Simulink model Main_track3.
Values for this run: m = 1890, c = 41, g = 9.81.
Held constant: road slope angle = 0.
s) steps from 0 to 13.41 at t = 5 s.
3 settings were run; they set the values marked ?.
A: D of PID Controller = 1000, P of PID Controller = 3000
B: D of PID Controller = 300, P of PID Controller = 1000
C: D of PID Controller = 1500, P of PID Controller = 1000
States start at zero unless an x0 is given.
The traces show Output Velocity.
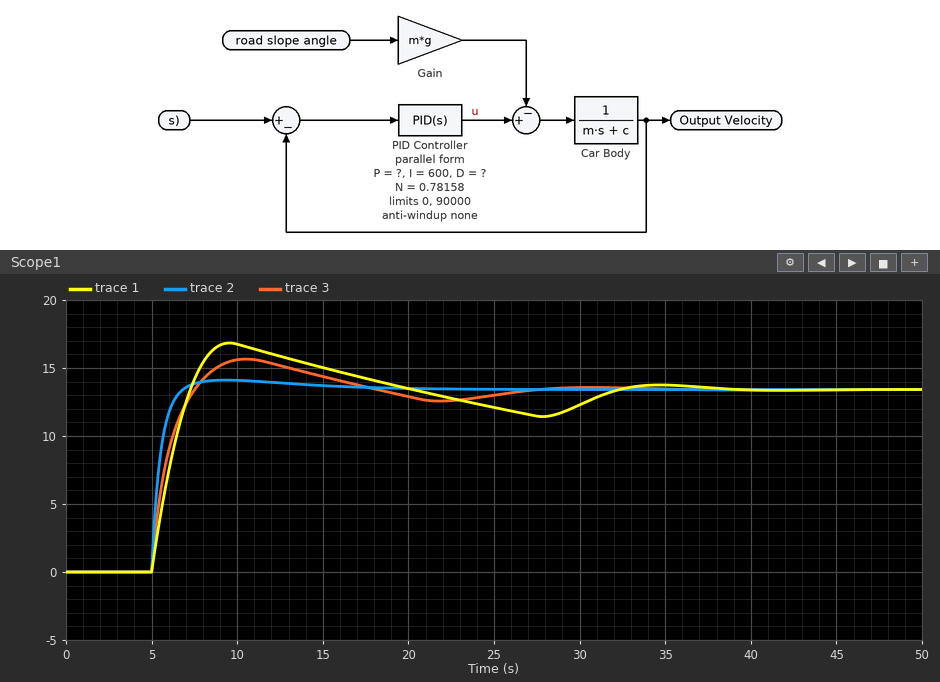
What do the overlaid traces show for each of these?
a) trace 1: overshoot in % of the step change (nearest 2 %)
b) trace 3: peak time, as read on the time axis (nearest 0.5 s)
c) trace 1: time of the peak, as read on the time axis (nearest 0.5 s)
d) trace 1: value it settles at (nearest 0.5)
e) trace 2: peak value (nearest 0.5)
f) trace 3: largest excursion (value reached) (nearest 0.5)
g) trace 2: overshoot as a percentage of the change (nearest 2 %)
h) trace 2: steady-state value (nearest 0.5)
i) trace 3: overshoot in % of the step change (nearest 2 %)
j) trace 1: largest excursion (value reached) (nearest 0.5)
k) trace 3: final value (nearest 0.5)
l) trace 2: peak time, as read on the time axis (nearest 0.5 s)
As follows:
26 %
10.5 s
9.5 s
13.5
14.0
15.5
6 %
13.5
16 %
17.0
13.5
9.5 s
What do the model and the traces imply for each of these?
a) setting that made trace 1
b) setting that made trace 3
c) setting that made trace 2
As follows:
B
C
A
